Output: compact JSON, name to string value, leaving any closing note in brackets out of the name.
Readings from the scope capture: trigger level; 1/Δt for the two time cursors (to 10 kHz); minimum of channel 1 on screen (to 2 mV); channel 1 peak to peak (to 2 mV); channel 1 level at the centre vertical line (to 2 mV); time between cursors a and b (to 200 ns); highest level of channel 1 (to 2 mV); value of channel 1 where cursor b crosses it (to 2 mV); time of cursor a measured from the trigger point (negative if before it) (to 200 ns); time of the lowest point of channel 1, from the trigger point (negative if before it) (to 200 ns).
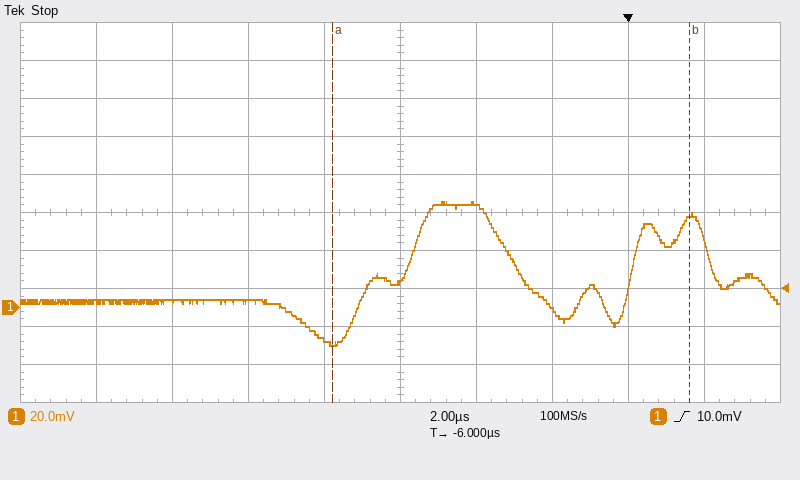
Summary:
{"trigger level": "10.0 mV", "1/Δt for the two time cursors": "110 kHz", "minimum of channel 1 on screen": "-20 mV", "channel 1 peak to peak": "76 mV", "channel 1 level at the centre vertical line": "14 mV", "time between cursors a and b": "9.4 µs", "highest level of channel 1": "56 mV", "value of channel 1 where cursor b crosses it": "48 mV", "time of cursor a measured from the trigger point (negative if before it)": "-7.8 µs", "time of the lowest point of channel 1, from the trigger point (negative if before it)": "-7.8 µs"}
